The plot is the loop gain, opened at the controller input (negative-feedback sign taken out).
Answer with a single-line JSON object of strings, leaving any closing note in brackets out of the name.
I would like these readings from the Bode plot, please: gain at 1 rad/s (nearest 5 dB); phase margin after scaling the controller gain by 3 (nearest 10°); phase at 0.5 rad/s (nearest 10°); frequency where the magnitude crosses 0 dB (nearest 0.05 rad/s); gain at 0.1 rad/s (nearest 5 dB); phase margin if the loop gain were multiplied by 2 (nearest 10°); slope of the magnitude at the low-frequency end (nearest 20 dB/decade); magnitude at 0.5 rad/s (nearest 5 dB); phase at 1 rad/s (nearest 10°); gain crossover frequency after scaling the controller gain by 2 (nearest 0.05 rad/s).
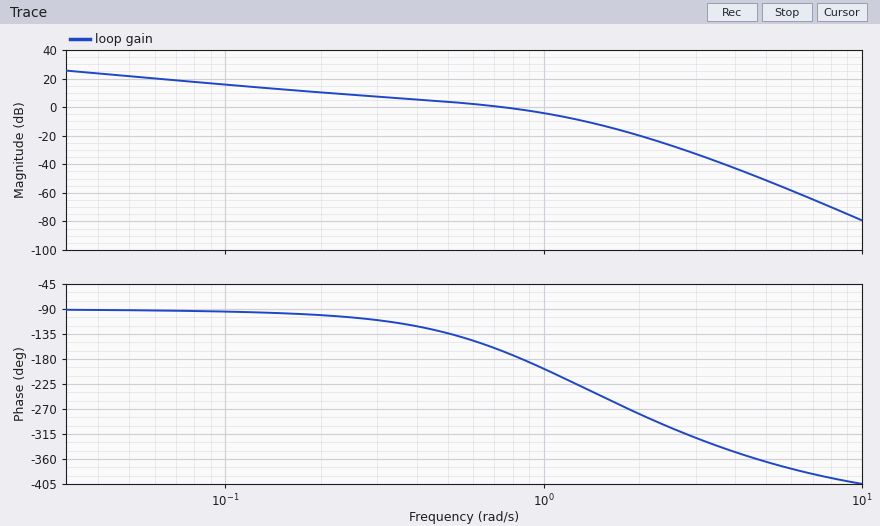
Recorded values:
{"gain at 1 rad/s": "-5 dB", "phase margin after scaling the controller gain by 3": "-50°", "phase at 0.5 rad/s": "-130°", "frequency where the magnitude crosses 0 dB": "0.75 rad/s", "gain at 0.1 rad/s": "15 dB", "phase margin if the loop gain were multiplied by 2": "-30°", "slope of the magnitude at the low-frequency end": "-20 dB/decade", "magnitude at 0.5 rad/s": "5 dB", "phase at 1 rad/s": "-200°", "gain crossover frequency after scaling the controller gain by 2": "1.10 rad/s"}
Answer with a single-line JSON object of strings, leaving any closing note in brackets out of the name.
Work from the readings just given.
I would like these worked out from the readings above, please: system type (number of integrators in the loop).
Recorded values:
{"system type": "1"}
